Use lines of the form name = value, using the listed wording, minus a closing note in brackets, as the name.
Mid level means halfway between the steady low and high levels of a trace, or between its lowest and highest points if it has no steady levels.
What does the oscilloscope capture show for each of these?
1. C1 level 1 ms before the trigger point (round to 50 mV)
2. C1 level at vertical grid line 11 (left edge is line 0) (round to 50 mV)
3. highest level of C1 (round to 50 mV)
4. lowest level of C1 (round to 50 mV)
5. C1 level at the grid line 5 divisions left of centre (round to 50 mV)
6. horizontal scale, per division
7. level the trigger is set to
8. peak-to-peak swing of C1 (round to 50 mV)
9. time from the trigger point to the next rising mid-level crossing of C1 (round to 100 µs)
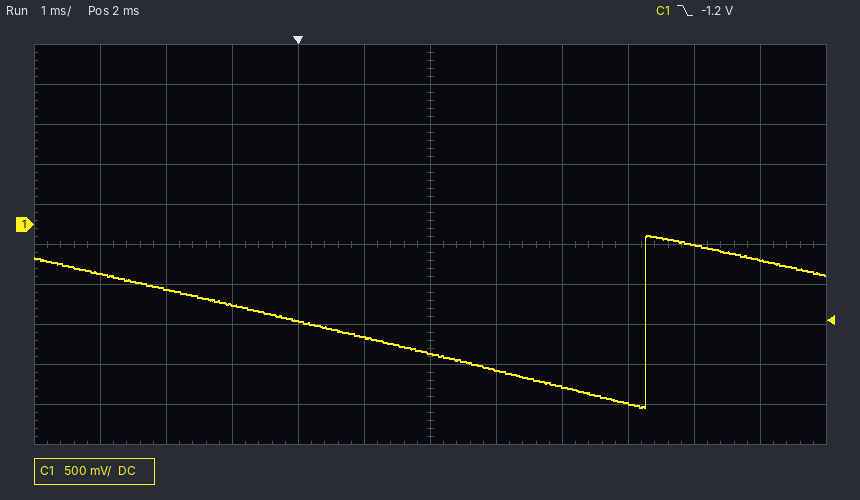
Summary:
C1 level 1 ms before the trigger point = -1.00 V
C1 level at vertical grid line 11 (left edge is line 0) = -450 mV
highest level of C1 = -150 mV
lowest level of C1 = -2.30 V
C1 level at the grid line 5 divisions left of centre = -600 mV
horizontal scale, per division = 1 ms
level the trigger is set to = -1.2 V
peak-to-peak swing of C1 = 2.15 V
time from the trigger point to the next rising mid-level crossing of C1 = 5.3 ms
